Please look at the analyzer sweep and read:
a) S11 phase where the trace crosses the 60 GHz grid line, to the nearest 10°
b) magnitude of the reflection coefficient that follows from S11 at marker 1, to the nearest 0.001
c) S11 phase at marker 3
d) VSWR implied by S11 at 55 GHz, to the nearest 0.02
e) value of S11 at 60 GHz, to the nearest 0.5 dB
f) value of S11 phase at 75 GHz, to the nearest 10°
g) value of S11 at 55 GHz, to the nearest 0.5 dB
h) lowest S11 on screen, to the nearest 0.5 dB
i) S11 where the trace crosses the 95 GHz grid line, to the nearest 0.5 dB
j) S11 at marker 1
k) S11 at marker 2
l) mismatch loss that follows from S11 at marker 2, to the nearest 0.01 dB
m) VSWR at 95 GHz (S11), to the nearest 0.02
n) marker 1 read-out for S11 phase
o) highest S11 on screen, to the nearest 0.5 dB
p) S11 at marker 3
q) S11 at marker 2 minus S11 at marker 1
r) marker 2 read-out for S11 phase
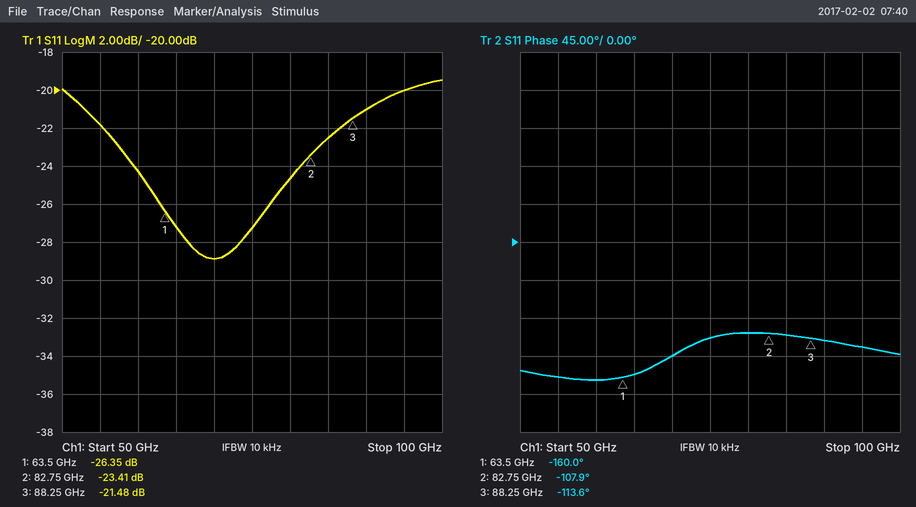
-160°
0.048
-113.6°
1.18
-24.5 dB
-110°
-22.0 dB
-29.0 dB
-20.0 dB
-26.35 dB
-23.41 dB
0.02 dB
1.22
-160.0°
-19.5 dB
-21.48 dB
2.94 dB
-107.9°
